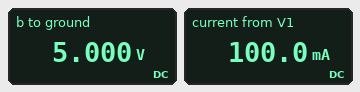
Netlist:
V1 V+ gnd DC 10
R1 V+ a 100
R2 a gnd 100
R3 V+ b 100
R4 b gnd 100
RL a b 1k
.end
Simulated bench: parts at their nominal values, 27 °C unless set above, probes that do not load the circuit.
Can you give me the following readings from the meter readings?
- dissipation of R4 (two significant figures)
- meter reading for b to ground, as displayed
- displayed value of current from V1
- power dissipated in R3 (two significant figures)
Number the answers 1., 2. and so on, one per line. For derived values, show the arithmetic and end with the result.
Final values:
1. (5 V)^2 / 100 Ω = 250 mW
2. 5.000 V
3. 100.0 mA
4. (10 V - 5 V)^2 / 100 Ω = 250 mW
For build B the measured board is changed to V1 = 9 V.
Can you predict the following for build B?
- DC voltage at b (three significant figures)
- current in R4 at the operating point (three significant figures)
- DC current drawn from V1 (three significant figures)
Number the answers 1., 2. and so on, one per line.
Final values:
1. 4.50 V
2. 45.0 mA
3. 90.0 mA
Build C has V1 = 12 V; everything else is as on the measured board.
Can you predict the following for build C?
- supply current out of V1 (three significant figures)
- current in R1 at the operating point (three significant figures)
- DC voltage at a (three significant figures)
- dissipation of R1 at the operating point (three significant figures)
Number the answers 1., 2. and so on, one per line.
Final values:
1. 120 mA
2. 60.0 mA
3. 6.00 V
4. 360 mW
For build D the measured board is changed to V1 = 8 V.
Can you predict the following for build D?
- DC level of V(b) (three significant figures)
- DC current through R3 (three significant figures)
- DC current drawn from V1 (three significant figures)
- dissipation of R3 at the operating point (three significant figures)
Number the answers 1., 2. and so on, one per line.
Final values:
1. 4.00 V
2. 40.0 mA
3. 80.0 mA
4. 160 mW
